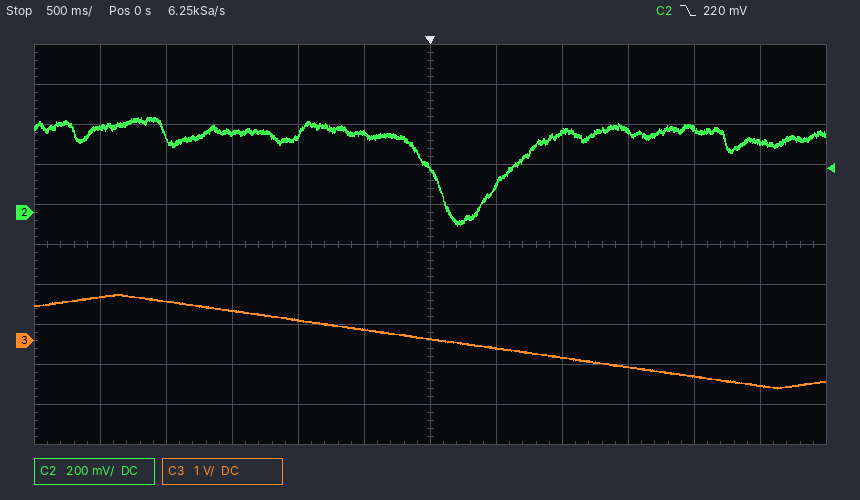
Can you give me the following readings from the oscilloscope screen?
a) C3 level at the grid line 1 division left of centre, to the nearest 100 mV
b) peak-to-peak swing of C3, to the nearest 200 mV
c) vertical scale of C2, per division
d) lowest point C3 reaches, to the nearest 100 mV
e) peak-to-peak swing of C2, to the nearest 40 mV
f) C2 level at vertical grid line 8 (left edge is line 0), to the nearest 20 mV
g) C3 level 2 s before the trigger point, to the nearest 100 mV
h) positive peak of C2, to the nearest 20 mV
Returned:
300 mV
2.4 V
200 mV
-1.2 V
560 mV
400 mV
1.0 V
480 mV
